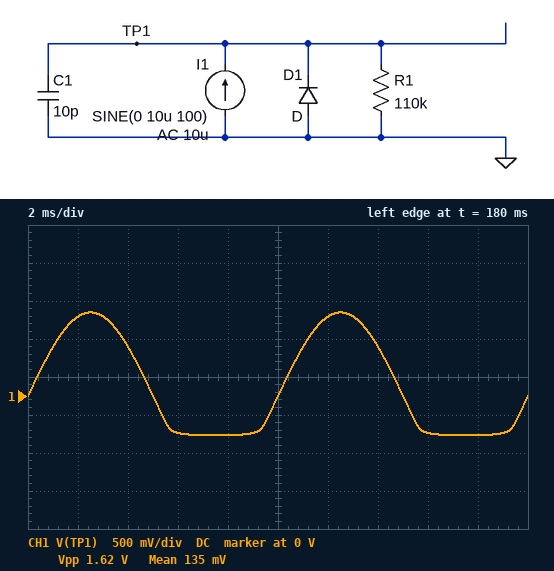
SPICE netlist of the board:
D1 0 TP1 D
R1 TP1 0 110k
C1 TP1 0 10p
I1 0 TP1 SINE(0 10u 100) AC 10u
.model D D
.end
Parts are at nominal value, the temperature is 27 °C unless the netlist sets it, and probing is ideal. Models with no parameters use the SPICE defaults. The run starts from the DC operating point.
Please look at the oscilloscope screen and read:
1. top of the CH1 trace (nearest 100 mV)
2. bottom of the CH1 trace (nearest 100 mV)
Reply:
1.1 V
-500 mV
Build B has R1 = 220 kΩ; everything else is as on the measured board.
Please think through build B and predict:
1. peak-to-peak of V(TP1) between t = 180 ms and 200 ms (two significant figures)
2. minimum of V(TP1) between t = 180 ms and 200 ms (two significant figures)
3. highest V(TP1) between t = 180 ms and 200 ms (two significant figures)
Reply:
2.7 V
-530 mV
2.2 V
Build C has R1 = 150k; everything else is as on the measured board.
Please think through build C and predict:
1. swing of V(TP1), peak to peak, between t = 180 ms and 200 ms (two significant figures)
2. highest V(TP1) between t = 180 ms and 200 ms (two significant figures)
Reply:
2.0 V
1.5 V
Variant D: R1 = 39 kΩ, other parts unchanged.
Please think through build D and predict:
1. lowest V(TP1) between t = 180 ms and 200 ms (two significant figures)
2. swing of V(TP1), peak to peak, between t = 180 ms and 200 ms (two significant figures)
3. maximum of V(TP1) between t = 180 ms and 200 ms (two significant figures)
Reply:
-390 mV
780 mV
390 mV
